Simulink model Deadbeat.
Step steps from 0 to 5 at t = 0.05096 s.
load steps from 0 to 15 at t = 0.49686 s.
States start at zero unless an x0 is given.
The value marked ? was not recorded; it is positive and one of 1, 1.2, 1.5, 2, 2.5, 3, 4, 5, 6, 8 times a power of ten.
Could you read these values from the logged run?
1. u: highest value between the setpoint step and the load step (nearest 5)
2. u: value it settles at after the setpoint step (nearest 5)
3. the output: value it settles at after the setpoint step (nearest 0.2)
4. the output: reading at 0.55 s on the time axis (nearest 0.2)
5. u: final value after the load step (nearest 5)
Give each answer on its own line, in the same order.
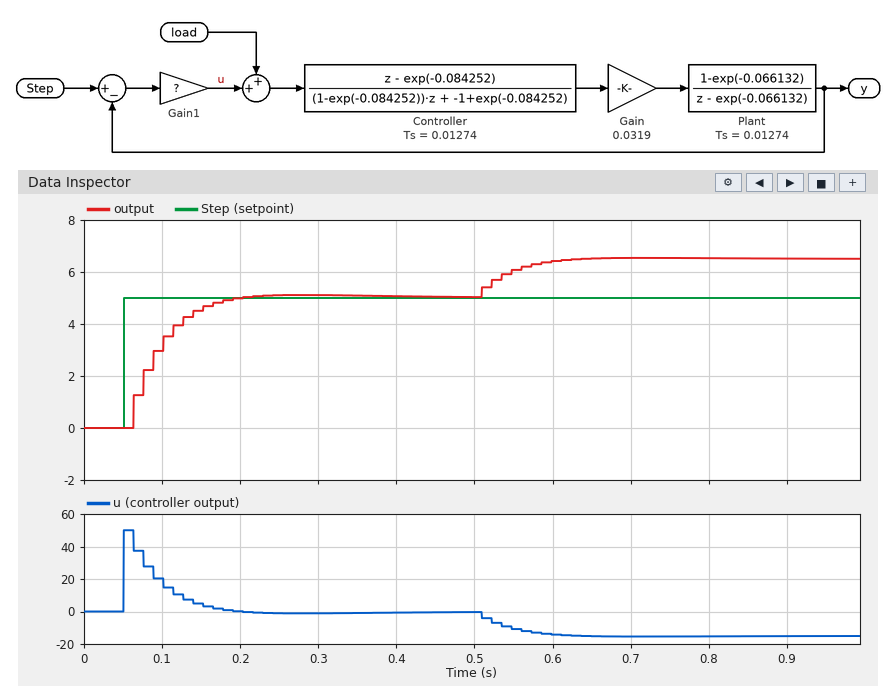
50
0
5.0
6.0
-15
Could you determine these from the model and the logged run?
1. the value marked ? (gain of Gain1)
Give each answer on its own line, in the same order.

10
